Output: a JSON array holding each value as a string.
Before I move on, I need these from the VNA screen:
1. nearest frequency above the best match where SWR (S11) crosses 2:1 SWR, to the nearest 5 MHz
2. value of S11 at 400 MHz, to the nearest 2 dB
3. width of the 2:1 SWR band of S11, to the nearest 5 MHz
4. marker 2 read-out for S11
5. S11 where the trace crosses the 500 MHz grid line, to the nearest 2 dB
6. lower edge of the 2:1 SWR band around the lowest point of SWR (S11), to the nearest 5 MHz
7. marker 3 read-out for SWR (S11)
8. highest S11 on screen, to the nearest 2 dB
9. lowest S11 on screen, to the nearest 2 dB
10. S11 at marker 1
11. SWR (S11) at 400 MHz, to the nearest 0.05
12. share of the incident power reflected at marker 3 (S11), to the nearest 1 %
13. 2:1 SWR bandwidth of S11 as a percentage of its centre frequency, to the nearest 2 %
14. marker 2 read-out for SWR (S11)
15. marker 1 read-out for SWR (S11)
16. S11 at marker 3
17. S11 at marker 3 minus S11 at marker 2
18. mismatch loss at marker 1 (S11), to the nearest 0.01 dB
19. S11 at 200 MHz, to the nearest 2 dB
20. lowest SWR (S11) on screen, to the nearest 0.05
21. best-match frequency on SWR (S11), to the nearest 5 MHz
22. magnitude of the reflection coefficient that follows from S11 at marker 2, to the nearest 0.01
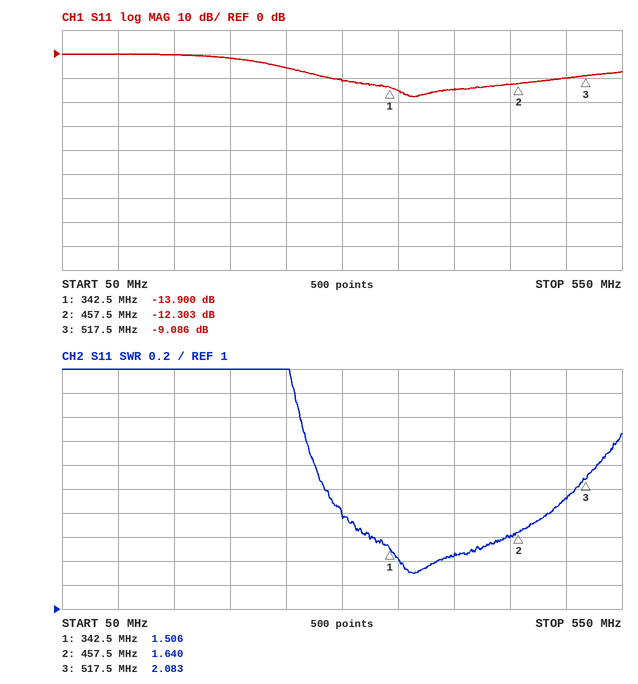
["510 MHz", "-14 dB", "225 MHz", "-12.303 dB", "-10 dB", "285 MHz", "2.083", "0 dB", "-18 dB", "-13.900 dB", "1.45", "12 %", "56 %", "1.640", "1.506", "-9.086 dB", "3.217 dB", "0.18 dB", "-2 dB", "1.30", "365 MHz", "0.24"]
